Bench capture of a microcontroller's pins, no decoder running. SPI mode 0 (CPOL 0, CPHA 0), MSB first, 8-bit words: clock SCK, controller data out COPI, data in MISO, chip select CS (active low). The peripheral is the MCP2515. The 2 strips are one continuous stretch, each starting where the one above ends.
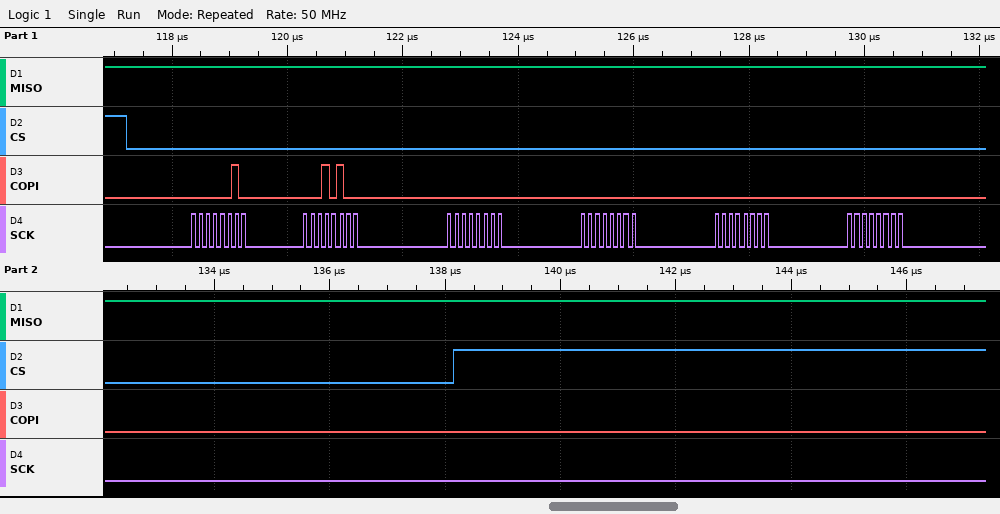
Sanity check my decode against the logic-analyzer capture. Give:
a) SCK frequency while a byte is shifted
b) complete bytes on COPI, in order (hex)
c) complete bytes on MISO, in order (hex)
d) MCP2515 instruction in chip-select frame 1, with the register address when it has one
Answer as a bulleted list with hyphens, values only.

- 8 MHz
- 02 14 00 00 00 00
- FF FF FF FF FF FF
- WRITE 0x14
